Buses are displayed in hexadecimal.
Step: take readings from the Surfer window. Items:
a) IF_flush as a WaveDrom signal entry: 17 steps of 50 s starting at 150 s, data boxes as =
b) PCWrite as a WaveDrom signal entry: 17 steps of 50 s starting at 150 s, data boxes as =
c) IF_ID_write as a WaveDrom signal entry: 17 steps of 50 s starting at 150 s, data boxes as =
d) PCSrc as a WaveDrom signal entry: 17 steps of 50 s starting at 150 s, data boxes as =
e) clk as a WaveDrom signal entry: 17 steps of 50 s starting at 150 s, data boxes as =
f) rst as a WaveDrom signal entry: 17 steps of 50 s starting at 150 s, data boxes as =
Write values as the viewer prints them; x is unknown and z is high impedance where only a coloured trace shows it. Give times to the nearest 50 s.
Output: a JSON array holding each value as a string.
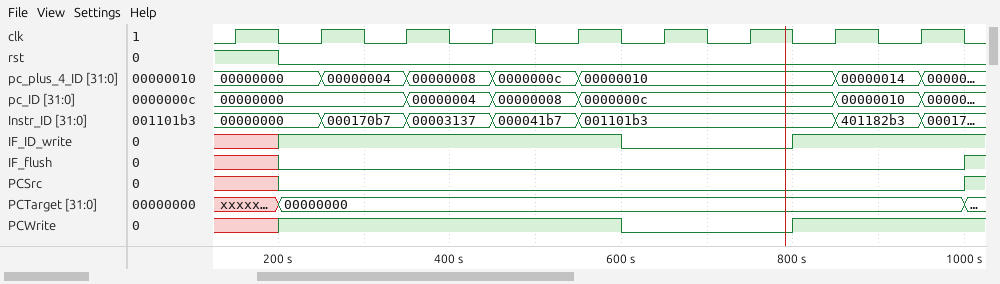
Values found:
["{name: 'IF_flush', wave: 'x0...............'}", "{name: 'PCWrite', wave: 'x1.......0...1...'}", "{name: 'IF_ID_write', wave: 'x1.......0...1...'}", "{name: 'PCSrc', wave: 'x0...............'}", "{name: 'clk', wave: '10101010101010101'}", "{name: 'rst', wave: '10...............'}"]
